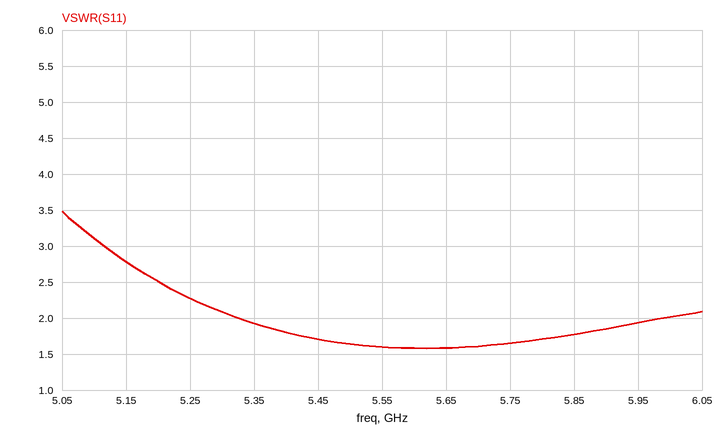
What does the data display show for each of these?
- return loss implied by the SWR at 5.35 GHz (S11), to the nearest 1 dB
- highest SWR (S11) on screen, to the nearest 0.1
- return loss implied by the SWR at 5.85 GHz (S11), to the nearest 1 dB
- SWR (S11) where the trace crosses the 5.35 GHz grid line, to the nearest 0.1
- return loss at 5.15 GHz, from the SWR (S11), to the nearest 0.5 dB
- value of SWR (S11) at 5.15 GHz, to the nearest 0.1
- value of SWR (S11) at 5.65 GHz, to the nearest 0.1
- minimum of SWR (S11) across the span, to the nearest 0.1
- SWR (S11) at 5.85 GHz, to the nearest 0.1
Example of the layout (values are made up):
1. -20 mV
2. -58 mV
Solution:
1. 10 dB
2. 3.5
3. 11 dB
4. 1.9
5. 6.5 dB
6. 2.8
7. 1.6
8. 1.6
9. 1.8
